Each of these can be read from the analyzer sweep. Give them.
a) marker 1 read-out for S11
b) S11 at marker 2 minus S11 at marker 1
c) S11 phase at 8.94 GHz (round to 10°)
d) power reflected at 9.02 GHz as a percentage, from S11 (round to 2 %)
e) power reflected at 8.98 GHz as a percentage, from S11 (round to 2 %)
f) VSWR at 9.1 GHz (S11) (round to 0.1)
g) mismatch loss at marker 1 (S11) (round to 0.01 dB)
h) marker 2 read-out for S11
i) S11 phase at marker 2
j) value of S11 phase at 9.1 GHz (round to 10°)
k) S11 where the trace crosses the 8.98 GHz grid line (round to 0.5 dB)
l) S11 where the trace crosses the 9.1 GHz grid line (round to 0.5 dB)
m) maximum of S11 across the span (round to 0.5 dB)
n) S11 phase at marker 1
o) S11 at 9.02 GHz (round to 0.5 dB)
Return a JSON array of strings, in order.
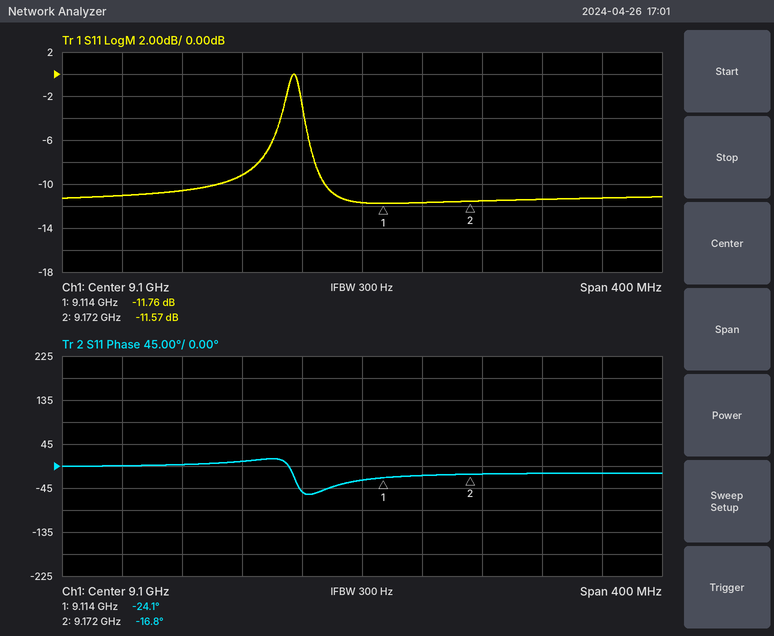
["-11.76 dB", "0.19 dB", "0°", "12 %", "8 %", "1.7", "0.30 dB", "-11.57 dB", "-16.8°", "-30°", "-10.5 dB", "-11.5 dB", "0.0 dB", "-24.1°", "-9.0 dB"]
